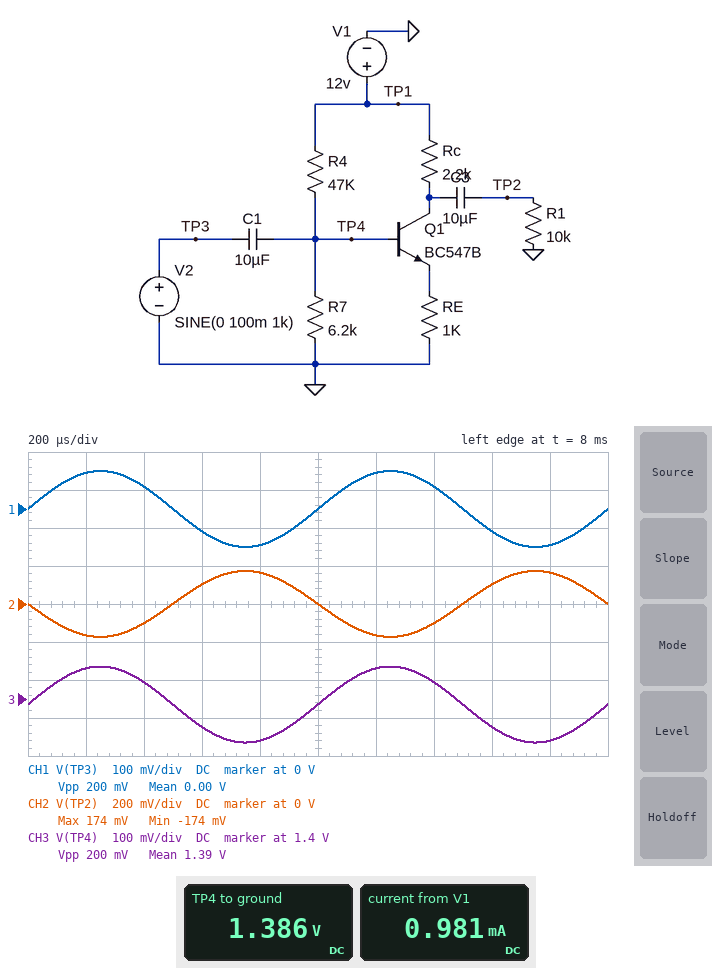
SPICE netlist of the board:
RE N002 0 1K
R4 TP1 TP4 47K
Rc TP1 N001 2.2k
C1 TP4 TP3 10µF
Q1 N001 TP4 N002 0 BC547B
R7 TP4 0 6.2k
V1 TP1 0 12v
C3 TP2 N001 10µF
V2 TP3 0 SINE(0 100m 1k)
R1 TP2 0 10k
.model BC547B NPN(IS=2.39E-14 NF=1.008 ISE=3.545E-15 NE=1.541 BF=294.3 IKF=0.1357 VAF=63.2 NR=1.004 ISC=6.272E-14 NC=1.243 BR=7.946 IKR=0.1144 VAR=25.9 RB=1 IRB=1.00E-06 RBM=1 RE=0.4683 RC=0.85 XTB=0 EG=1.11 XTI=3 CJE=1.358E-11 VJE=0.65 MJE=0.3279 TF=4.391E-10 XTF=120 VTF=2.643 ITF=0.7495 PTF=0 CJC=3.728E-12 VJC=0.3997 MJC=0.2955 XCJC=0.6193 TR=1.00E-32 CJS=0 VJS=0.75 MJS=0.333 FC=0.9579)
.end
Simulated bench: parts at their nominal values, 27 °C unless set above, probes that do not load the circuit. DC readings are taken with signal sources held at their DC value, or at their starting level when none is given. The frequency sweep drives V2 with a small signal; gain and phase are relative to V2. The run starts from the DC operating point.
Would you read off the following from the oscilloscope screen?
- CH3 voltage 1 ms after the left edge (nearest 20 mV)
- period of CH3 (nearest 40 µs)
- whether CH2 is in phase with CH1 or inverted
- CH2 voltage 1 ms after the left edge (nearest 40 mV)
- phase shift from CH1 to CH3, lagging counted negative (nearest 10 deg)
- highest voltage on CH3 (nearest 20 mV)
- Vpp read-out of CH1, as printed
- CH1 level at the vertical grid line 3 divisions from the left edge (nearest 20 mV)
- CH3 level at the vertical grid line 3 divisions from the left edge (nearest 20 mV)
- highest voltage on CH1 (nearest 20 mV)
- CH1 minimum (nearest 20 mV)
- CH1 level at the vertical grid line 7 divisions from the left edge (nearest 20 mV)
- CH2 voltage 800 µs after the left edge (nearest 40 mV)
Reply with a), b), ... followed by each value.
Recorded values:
a) 1.38 V
b) 1.00 ms
c) inverted
d) 0 V
e) 0 deg
f) 1.48 V
g) 200 mV
h) -60 mV
i) 1.32 V
j) 100 mV
k) -100 mV
l) 60 mV
m) 160 mV
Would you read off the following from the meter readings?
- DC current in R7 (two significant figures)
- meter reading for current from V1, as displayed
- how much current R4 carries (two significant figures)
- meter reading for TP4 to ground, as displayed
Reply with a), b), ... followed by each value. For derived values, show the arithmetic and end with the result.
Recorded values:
a) (1.386 V) / 6.2 kΩ = 220 µA
b) 0.981 mA
c) (12 V - 1.386 V) / 47 kΩ = 230 µA
d) 1.386 V
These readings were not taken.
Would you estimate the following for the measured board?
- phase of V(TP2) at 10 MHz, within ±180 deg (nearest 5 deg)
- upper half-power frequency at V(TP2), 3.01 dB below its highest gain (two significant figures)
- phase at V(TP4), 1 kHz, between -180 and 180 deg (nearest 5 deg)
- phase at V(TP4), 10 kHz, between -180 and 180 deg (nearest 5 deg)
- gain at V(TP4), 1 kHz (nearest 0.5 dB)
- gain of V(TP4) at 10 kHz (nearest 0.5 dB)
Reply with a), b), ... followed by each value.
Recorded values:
a) 160 deg
b) 150 MHz
c) 0 deg
d) 0 deg
e) 0 dB
f) 0 dB
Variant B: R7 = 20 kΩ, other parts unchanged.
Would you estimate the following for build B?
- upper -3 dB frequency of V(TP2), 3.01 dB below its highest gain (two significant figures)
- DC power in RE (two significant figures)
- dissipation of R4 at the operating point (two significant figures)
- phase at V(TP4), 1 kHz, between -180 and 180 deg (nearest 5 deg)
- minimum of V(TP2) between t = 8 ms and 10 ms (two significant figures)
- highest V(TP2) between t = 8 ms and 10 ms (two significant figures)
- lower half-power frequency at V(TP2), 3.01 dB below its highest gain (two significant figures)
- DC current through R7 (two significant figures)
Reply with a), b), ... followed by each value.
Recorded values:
a) 130 MHz
b) 7.7 mW
c) 1.6 mW
d) 0 deg
e) -180 mV
f) 180 mV
g) 1.9 Hz
h) 170 µA
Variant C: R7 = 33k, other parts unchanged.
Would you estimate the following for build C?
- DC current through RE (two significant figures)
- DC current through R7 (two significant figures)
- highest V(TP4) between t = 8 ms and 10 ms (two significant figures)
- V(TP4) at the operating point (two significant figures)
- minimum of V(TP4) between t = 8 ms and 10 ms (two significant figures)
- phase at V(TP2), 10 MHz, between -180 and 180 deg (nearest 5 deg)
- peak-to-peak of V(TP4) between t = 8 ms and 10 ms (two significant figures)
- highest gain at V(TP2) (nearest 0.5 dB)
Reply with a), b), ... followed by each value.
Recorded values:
a) 3.7 mA
b) 130 µA
c) 4.5 V
d) 4.4 V
e) 4.3 V
f) 30 deg
g) 200 mV
h) 0 dB
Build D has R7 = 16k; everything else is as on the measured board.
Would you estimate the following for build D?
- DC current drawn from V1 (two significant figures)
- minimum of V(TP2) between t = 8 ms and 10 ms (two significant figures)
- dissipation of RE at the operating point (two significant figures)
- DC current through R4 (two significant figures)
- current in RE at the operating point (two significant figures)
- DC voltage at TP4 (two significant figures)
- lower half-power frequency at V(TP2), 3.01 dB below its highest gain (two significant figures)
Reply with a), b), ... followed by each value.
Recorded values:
a) 2.5 mA
b) -180 mV
c) 5.3 mW
d) 190 µA
e) 2.3 mA
f) 3.0 V
g) 2.1 Hz
